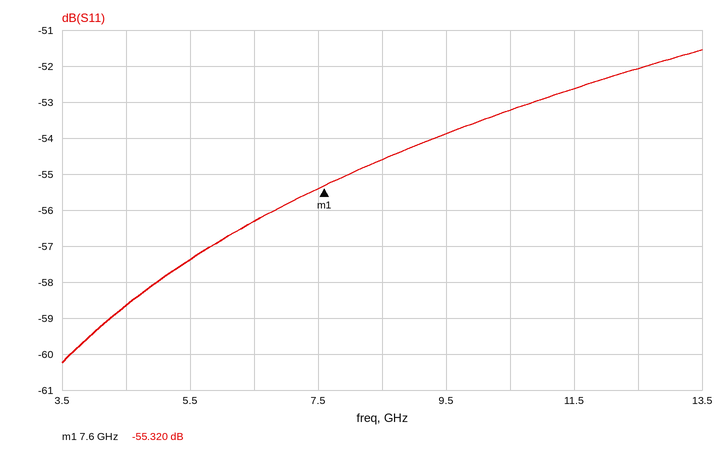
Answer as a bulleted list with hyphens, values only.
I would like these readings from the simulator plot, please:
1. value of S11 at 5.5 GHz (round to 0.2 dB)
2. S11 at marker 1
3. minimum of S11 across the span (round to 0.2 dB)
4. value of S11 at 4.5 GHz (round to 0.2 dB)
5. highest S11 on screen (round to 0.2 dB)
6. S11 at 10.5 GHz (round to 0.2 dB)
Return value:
- -57.4 dB
- -55.320 dB
- -60.2 dB
- -58.6 dB
- -51.6 dB
- -53.2 dB
